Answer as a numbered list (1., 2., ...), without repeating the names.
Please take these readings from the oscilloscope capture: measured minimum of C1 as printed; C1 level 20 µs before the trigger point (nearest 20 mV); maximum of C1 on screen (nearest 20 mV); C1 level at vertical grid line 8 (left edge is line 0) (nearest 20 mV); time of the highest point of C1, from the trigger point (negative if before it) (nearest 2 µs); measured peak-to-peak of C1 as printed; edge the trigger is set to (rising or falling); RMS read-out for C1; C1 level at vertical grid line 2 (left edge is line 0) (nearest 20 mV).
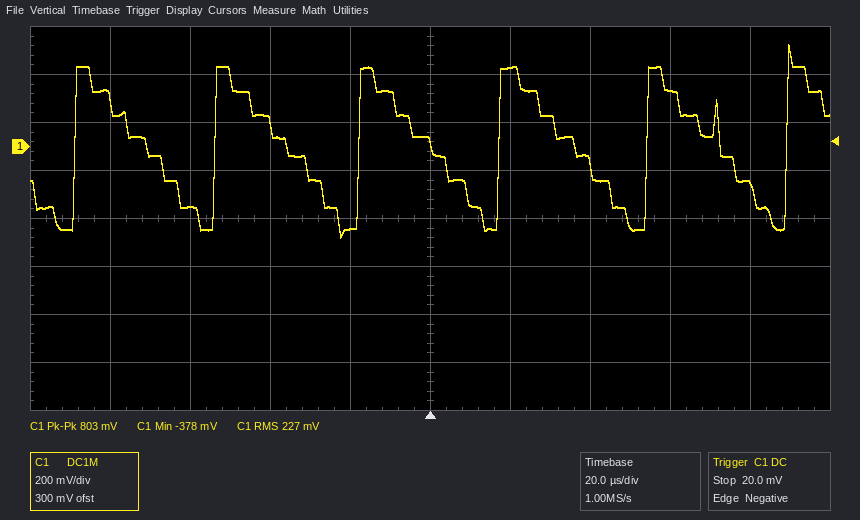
1. -378 mV
2. -340 mV
3. 420 mV
4. 240 mV
5. +90 µs
6. 803 mV
7. falling
8. 227 mV
9. -260 mV
